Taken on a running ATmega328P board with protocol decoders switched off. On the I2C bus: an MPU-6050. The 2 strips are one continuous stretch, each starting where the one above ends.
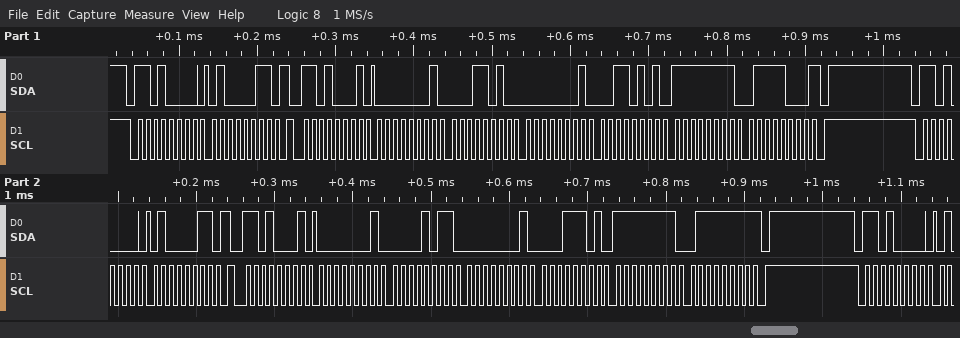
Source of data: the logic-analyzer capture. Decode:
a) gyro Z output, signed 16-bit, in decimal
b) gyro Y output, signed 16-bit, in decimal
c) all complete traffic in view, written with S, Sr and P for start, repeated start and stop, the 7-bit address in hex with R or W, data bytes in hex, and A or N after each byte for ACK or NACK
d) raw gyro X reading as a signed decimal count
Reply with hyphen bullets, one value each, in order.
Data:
- -136
- 309
- S 68W A 43 A Sr 68R A 01 A 1A A 01 A 35 A FF A 78 N P S 68W A 43 A Sr 68R A 01 A 0B A 01 A 1D A FF A 7F N P S 68W A
- 282
